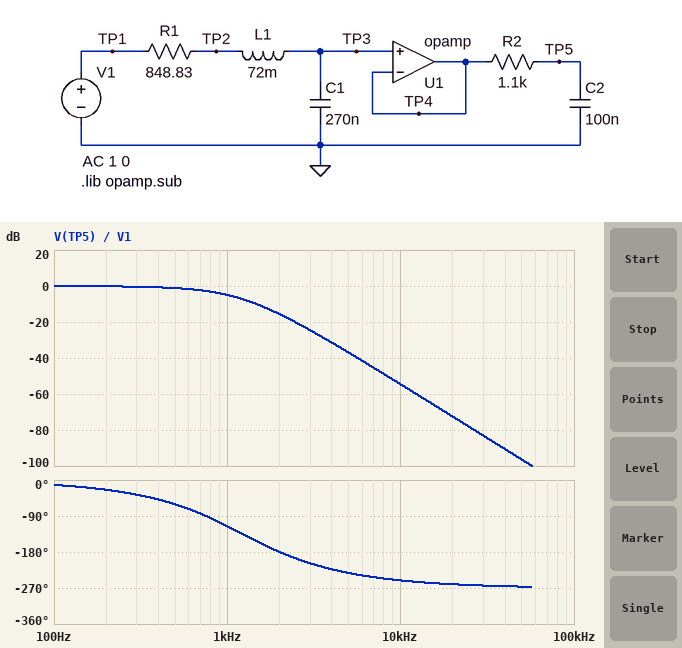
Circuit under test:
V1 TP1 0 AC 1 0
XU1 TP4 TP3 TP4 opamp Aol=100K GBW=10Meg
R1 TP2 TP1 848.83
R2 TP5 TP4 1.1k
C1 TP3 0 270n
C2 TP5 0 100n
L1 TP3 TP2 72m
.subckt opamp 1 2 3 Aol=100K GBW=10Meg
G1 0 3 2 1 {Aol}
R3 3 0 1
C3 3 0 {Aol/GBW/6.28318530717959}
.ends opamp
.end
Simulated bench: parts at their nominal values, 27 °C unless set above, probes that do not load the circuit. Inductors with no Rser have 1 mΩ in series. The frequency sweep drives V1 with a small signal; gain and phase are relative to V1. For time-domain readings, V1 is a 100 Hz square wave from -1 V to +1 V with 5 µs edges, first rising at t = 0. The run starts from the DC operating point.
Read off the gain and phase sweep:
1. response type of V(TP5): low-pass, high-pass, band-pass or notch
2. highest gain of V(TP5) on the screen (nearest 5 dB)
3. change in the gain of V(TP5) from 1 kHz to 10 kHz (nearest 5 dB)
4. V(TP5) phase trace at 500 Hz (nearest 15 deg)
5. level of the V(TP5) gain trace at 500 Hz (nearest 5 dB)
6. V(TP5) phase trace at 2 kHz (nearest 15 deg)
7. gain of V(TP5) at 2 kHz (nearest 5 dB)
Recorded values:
low-pass
0 dB
-50 dB
-60 deg
0 dB
-180 deg
-15 dB
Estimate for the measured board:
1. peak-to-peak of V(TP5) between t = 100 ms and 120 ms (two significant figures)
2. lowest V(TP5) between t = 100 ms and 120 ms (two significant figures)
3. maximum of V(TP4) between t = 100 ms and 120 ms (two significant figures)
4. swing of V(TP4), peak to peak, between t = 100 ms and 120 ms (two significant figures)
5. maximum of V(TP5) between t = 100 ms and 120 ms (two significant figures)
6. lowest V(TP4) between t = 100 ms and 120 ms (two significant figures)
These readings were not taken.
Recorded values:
2.0 V
-1.0 V
1.0 V
2.0 V
1.0 V
-1.0 V
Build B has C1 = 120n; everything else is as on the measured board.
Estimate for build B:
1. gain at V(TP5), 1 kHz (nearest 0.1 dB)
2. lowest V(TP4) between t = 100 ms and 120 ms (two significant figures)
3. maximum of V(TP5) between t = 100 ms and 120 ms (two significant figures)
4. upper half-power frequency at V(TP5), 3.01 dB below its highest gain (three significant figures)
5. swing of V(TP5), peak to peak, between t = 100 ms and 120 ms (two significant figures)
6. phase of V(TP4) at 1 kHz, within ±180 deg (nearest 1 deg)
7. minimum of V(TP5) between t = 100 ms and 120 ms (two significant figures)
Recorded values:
-1.0 dB
-1.3 V
1.1 V
1.49 kHz
2.2 V
-44 deg
-1.1 V
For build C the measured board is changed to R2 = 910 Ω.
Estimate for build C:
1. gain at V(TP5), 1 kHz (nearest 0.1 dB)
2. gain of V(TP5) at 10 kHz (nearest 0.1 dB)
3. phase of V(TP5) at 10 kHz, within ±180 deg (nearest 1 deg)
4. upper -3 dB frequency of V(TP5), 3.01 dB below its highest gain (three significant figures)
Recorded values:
-4.5 dB
-53.0 dB
111 deg
824 Hz
